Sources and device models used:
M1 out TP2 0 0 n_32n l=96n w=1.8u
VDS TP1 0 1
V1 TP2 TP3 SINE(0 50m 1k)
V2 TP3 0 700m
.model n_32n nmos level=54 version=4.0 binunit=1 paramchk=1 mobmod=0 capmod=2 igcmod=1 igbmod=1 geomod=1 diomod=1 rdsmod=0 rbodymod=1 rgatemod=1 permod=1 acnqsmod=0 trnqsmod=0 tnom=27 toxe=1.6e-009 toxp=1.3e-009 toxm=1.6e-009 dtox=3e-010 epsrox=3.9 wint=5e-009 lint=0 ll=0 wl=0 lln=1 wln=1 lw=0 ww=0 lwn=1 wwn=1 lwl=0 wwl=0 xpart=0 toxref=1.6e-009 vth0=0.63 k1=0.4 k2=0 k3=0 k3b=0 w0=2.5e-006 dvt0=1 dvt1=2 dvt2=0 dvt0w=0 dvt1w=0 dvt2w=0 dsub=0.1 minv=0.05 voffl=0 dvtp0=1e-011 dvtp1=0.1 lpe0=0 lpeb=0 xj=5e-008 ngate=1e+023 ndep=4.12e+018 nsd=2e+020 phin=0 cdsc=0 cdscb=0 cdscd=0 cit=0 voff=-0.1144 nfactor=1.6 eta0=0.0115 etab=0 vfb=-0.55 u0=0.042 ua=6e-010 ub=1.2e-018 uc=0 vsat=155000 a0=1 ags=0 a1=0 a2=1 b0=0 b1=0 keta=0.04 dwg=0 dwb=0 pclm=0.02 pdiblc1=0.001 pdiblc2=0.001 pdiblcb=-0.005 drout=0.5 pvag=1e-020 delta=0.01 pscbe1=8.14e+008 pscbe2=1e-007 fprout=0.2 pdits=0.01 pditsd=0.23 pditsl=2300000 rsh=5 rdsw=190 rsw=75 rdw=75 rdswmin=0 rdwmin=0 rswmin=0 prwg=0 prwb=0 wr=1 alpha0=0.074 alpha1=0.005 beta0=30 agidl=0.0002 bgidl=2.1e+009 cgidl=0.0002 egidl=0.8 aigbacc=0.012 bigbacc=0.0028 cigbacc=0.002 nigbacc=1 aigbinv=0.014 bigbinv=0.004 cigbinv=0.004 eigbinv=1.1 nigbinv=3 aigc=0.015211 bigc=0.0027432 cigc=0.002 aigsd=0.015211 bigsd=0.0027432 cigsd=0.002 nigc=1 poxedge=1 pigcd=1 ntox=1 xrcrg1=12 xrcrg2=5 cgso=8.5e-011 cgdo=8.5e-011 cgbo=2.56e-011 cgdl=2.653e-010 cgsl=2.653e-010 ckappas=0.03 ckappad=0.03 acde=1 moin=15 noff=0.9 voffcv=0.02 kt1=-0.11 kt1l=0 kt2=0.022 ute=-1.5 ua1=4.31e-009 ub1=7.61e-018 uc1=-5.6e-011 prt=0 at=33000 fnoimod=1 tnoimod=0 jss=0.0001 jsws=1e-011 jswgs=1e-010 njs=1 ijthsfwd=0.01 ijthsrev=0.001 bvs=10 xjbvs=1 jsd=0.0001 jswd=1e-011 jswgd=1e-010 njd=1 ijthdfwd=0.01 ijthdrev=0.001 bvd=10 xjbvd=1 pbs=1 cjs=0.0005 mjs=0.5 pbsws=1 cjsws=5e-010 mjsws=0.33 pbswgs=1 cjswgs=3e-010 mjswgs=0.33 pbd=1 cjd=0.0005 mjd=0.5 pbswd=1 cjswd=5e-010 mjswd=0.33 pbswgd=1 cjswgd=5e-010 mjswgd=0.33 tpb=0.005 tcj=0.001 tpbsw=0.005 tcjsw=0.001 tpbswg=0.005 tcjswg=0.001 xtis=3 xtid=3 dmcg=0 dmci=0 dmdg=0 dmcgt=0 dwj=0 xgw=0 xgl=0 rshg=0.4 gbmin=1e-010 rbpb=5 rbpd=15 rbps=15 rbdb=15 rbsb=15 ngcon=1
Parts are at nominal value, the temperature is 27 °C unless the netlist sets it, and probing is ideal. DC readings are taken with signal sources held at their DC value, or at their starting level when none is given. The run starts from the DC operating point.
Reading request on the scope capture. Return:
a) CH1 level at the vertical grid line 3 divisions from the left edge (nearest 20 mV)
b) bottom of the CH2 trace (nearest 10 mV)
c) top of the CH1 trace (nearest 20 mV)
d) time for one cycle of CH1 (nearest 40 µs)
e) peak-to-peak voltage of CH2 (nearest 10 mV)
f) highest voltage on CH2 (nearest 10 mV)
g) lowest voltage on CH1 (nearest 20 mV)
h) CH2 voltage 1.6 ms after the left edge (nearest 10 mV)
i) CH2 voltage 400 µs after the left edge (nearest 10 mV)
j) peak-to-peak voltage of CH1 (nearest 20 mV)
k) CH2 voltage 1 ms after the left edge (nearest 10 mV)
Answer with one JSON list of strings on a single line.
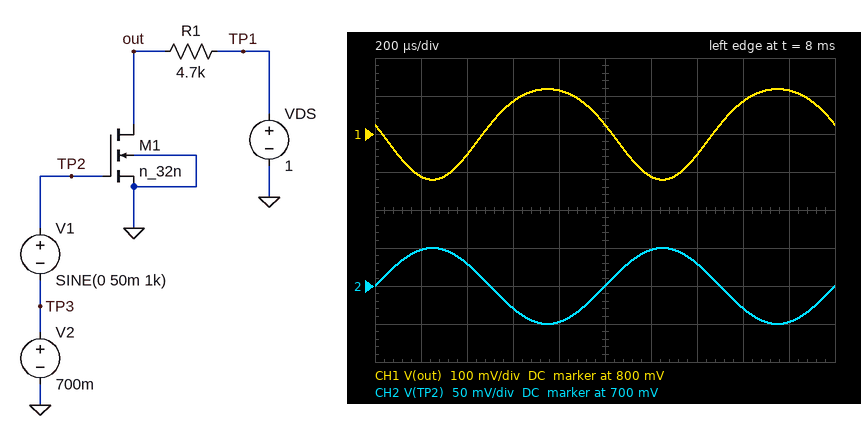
["880 mV", "650 mV", "920 mV", "1.00 ms", "100 mV", "750 mV", "680 mV", "670 mV", "730 mV", "240 mV", "700 mV"]
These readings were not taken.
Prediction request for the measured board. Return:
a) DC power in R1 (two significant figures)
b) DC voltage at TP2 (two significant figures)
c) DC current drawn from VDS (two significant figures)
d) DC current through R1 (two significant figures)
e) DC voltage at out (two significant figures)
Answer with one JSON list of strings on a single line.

["6.6 µW", "700 mV", "37 µA", "37 µA", "820 mV"]
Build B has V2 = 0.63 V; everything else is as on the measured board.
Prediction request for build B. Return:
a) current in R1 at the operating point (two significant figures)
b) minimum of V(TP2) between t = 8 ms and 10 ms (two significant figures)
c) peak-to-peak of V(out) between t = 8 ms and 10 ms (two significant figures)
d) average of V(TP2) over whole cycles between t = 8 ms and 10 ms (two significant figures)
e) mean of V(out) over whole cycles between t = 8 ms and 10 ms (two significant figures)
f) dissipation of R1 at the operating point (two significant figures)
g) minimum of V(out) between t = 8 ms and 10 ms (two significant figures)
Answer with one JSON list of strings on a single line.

["12 µA", "580 mV", "110 mV", "630 mV", "930 mV", "710 nW", "870 mV"]
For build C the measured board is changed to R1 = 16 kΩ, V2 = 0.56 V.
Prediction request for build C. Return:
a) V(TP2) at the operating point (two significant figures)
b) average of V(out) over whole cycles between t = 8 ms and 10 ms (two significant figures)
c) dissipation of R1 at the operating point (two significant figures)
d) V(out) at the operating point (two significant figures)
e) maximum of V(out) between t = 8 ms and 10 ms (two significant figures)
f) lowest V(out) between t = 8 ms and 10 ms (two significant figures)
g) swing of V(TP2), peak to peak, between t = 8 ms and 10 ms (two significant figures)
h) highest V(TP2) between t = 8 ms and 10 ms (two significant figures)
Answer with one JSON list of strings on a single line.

["560 mV", "940 mV", "150 nW", "950 mV", "980 mV", "870 mV", "100 mV", "610 mV"]
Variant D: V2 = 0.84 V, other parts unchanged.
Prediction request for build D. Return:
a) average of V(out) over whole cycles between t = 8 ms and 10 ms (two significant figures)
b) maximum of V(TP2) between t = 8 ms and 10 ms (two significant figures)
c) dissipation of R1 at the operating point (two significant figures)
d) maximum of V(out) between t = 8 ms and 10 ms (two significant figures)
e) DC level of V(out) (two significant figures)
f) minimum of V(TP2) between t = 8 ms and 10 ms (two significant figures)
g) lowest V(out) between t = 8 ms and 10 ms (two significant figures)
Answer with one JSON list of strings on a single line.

["340 mV", "890 mV", "99 µW", "530 mV", "320 mV", "790 mV", "190 mV"]
